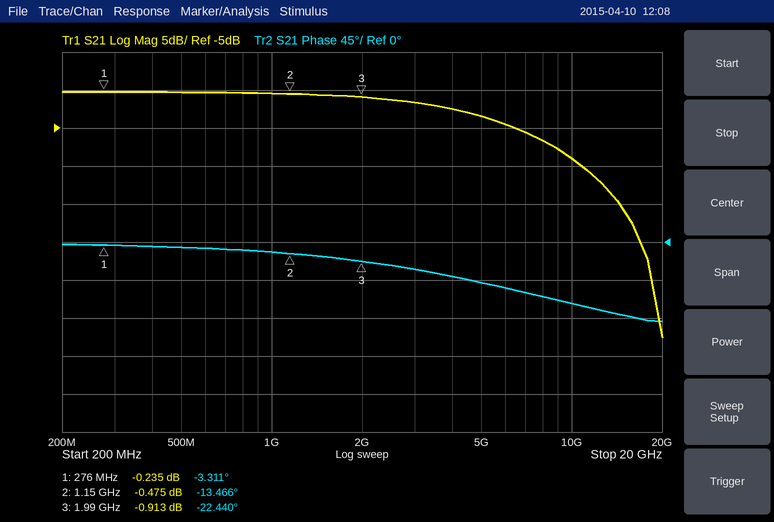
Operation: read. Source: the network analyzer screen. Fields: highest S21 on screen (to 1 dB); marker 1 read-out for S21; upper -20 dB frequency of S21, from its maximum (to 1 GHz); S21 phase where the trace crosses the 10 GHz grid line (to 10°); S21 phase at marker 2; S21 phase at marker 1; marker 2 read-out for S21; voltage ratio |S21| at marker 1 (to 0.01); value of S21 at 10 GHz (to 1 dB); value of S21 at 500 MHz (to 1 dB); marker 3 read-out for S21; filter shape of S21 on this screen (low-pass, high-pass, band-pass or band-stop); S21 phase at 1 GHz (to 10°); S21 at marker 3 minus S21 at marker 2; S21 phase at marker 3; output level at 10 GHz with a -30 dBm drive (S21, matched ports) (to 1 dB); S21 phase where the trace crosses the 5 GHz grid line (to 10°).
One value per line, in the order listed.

0 dB
-0.235 dB
17 GHz
-70°
-13.466°
-3.311°
-0.475 dB
0.97
-9 dB
0 dB
-0.913 dB
low-pass
-10°
-0.438 dB
-22.440°
-39 dBm
-50°
